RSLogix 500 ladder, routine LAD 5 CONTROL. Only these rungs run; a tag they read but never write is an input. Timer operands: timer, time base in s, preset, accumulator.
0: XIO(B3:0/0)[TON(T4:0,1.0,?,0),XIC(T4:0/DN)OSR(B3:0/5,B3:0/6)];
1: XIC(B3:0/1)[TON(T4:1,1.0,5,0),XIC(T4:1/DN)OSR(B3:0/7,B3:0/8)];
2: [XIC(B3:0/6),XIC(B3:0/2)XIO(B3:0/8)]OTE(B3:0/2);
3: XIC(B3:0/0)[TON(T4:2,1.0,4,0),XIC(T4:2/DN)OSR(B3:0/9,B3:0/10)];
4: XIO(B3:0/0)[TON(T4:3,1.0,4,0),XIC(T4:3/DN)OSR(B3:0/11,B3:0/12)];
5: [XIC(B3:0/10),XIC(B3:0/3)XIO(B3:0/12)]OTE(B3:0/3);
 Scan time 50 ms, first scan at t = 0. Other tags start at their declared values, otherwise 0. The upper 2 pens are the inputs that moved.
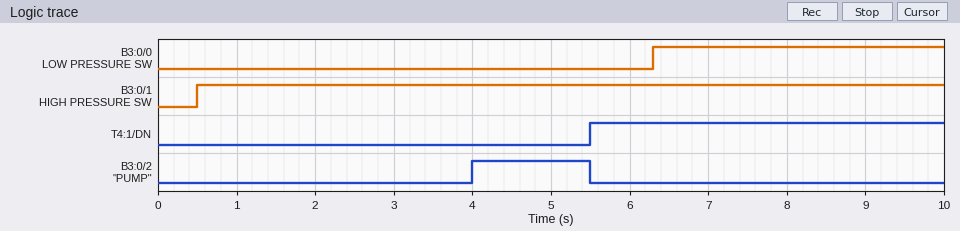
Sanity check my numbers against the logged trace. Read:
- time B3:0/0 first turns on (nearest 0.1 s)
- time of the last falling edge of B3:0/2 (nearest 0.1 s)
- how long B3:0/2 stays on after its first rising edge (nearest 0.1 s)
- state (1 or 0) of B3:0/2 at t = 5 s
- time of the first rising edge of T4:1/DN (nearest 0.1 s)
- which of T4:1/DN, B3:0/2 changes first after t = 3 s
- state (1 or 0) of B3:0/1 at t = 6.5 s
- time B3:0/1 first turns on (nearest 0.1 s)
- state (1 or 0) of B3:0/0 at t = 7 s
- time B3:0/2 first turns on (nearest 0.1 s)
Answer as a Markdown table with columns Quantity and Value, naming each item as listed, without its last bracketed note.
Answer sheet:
| Quantity | Value |
|---|---|
| time B3:0/0 first turns on | 6.3 s |
| time of the last falling edge of B3:0/2 | 5.5 s |
| how long B3:0/2 stays on after its first rising edge | 1.5 s |
| state (1 or 0) of B3:0/2 at t = 5 s | 1 |
| time of the first rising edge of T4:1/DN | 5.5 s |
| which of T4:1/DN, B3:0/2 changes first after t = 3 s | B3:0/2 |
| state (1 or 0) of B3:0/1 at t = 6.5 s | 1 |
| time B3:0/1 first turns on | 0.5 s |
| state (1 or 0) of B3:0/0 at t = 7 s | 1 |
| time B3:0/2 first turns on | 4.0 s |
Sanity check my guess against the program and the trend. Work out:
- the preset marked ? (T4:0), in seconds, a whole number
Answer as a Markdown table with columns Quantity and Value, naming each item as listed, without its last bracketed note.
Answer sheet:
| Quantity | Value |
|---|---|
| the preset marked ? (T4:0), in seconds, a whole number | 4 s |
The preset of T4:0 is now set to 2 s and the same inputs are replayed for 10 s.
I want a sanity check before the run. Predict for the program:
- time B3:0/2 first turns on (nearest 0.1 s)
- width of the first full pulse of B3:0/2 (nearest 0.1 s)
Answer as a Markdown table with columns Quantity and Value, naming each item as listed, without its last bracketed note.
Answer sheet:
| Quantity | Value |
|---|---|
| time B3:0/2 first turns on | 2.0 s |
| width of the first full pulse of B3:0/2 | 3.5 s |
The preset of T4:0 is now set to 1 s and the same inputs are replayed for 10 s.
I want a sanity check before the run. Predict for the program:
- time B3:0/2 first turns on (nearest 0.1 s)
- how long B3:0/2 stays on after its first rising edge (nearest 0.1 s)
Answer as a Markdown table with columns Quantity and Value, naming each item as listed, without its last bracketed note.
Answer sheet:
| Quantity | Value |
|---|---|
| time B3:0/2 first turns on | 1.0 s |
| how long B3:0/2 stays on after its first rising edge | 4.5 s |
